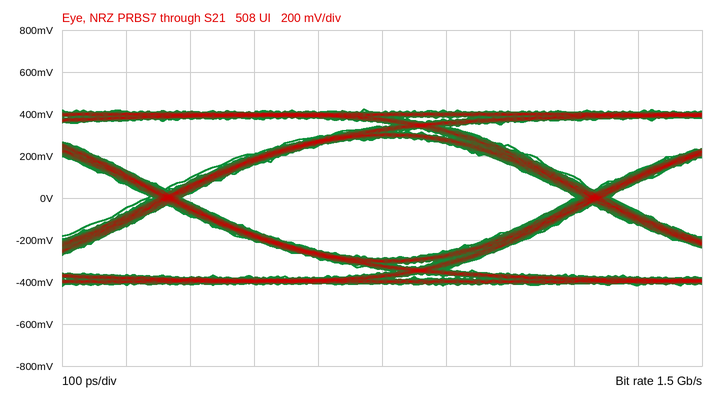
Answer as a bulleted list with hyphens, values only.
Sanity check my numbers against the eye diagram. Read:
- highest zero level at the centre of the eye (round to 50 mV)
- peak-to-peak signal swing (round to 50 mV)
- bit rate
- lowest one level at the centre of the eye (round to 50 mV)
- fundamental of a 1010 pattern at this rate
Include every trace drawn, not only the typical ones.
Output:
- -300 mV
- 850 mV
- 1.5 Gb/s
- 300 mV
- 750 MHz
